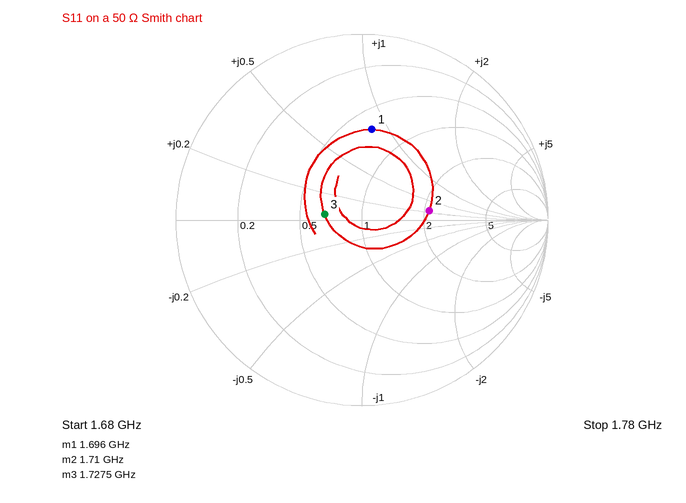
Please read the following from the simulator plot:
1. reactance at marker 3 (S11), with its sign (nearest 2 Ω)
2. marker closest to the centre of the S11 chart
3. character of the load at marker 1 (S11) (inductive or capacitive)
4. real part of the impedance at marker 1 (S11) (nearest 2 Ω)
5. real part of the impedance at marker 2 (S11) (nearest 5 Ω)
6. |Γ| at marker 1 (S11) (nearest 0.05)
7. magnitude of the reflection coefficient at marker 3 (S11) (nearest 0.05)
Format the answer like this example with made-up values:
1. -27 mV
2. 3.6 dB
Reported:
1. +2 Ω
2. marker 3
3. inductive
4. 34 Ω
5. 105 Ω
6. 0.50
7. 0.20
